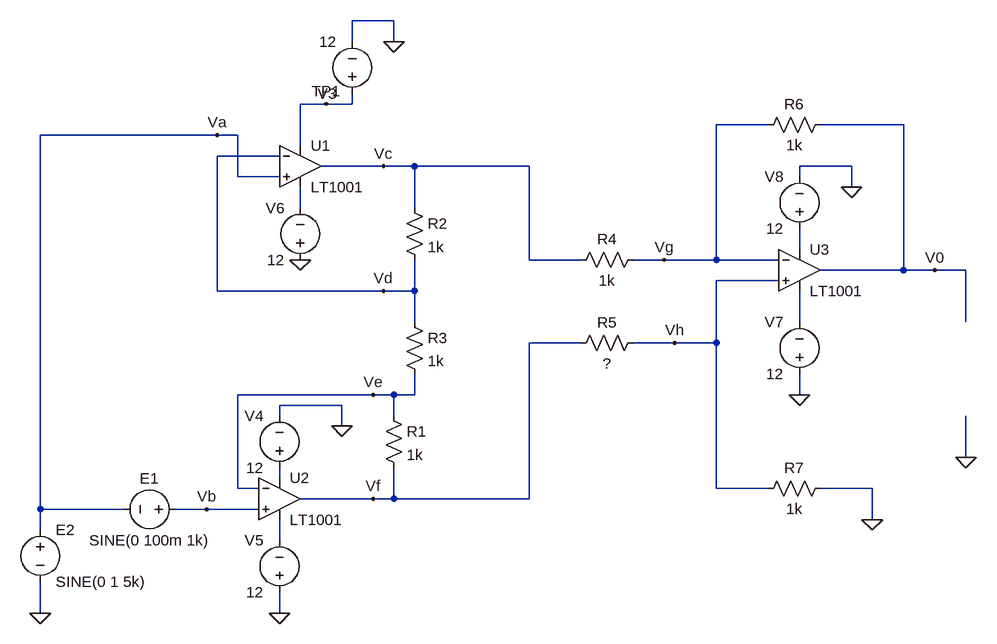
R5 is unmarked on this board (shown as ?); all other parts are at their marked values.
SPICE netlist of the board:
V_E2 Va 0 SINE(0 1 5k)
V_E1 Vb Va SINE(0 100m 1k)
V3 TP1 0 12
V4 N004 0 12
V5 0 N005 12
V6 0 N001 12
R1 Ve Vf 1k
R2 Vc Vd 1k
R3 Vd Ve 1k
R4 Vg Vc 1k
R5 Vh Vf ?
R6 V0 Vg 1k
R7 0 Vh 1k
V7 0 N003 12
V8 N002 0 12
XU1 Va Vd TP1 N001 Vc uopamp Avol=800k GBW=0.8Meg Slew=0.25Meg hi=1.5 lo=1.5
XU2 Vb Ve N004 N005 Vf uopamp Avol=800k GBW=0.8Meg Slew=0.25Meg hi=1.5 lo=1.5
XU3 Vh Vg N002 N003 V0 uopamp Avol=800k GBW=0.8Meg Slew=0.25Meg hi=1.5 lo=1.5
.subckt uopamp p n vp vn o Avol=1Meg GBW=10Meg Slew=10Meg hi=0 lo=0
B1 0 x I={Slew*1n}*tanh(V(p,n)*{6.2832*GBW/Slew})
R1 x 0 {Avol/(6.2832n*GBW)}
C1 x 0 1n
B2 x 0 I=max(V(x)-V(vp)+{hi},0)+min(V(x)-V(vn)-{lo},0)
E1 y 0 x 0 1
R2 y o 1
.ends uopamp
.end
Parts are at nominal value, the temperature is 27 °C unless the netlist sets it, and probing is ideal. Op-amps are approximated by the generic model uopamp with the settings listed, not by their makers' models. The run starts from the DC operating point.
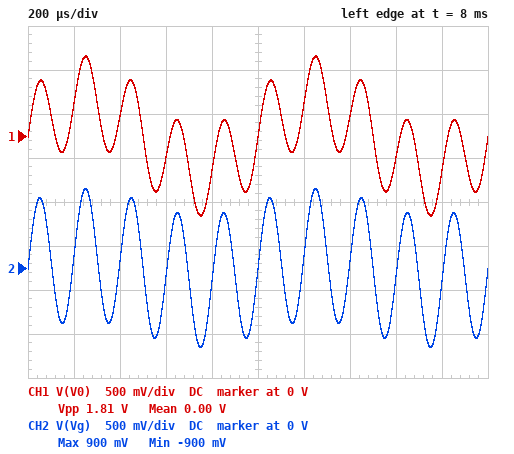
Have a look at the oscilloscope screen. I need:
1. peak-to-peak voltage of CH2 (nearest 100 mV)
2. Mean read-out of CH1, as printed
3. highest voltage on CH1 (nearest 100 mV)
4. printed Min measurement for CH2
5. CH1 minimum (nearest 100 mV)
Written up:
1.8 V
0.00 V
900 mV
-900 mV
-900 mV
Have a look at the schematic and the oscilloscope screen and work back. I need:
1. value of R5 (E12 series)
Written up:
330 Ω
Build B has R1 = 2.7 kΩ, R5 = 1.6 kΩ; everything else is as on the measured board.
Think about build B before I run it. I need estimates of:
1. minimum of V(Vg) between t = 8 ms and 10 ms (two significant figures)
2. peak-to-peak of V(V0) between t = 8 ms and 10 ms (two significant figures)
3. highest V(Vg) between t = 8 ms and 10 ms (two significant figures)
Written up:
-530 mV
1.1 V
530 mV
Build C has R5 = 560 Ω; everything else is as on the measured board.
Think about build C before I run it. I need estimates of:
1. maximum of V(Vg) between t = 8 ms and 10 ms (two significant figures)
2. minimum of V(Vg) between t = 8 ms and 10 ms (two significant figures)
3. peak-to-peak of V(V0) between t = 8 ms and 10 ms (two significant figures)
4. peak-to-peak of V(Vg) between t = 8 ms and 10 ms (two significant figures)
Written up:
770 mV
-770 mV
1.3 V
1.5 V
